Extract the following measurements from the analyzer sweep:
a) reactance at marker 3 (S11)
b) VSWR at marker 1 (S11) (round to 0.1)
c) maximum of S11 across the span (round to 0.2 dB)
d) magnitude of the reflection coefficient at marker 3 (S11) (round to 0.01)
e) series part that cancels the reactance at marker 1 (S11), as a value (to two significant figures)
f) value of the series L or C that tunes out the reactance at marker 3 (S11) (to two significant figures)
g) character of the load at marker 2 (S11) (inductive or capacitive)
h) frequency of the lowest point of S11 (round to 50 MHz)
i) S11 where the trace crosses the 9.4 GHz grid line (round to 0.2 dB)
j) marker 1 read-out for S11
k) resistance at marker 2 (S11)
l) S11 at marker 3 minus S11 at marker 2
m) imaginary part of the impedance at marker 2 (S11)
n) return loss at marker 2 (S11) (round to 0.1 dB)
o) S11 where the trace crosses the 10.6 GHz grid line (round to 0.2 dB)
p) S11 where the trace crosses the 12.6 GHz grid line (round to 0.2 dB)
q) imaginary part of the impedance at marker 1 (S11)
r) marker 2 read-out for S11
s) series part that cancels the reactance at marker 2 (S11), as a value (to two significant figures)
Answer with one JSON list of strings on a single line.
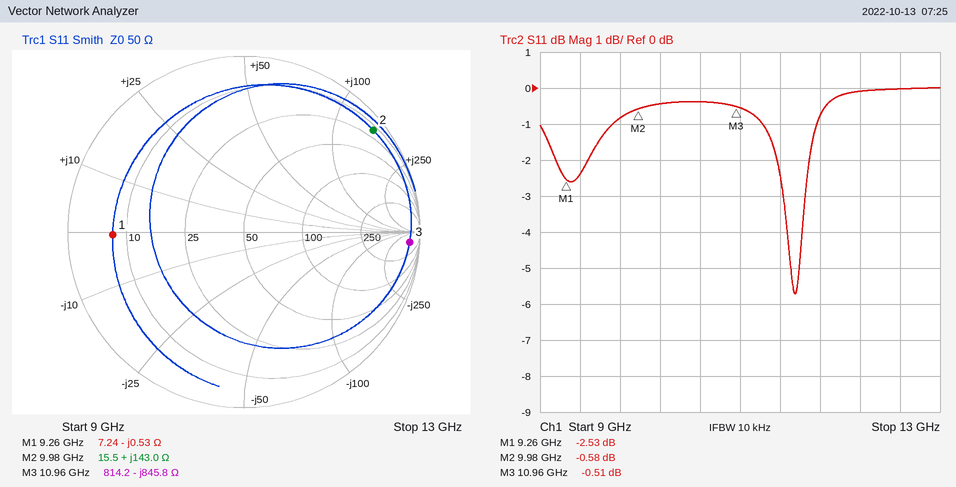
["-845.8 Ω", "6.9", "0.0 dB", "0.94", "9.1 pH", "12 nH", "inductive", "11.55 GHz", "-2.4 dB", "-2.53 dB", "15.5 Ω", "0.07 dB", "+143.0 Ω", "0.6 dB", "-0.4 dB", "0.0 dB", "-0.53 Ω", "-0.58 dB", "110 fF"]
